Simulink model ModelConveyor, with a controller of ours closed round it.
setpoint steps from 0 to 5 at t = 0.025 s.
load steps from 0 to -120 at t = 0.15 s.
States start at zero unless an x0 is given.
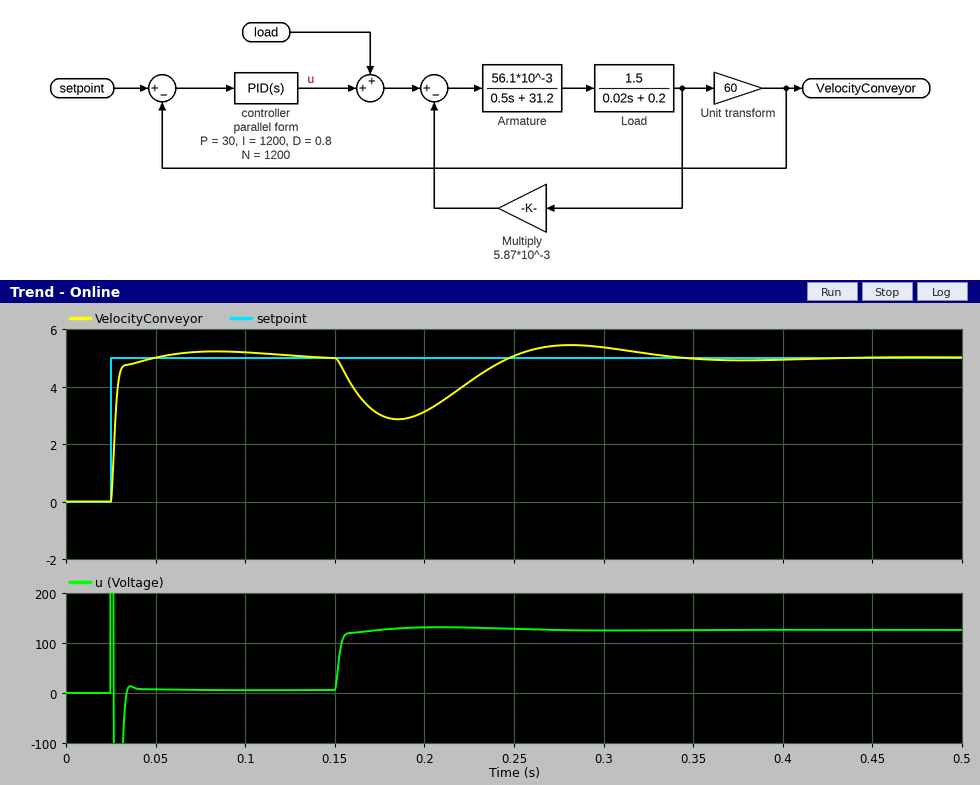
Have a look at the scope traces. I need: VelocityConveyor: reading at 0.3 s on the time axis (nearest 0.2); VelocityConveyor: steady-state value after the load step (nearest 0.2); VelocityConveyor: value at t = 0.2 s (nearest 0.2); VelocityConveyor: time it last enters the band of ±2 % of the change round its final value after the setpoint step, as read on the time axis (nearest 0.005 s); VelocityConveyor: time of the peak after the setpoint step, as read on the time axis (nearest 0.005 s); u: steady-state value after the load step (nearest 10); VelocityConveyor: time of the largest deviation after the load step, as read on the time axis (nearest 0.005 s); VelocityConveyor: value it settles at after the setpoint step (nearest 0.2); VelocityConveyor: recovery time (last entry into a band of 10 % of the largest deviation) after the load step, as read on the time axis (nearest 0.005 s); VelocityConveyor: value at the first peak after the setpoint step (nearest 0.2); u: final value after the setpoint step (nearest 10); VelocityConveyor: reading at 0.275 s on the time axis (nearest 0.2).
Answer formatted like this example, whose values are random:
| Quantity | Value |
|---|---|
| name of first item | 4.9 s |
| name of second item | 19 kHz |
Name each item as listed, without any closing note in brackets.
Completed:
| Quantity | Value |
|---|---|
| VelocityConveyor: reading at 0.3 s on the time axis | 5.4 |
| VelocityConveyor: steady-state value after the load step | 5.0 |
| VelocityConveyor: value at t = 0.2 s | 3.2 |
| VelocityConveyor: time it last enters the band of ±2 % of the change round its final value after the setpoint step, as read on the time axis | 0.120 s |
| VelocityConveyor: time of the peak after the setpoint step, as read on the time axis | 0.085 s |
| u: steady-state value after the load step | 130 |
| VelocityConveyor: time of the largest deviation after the load step, as read on the time axis | 0.185 s |
| VelocityConveyor: value it settles at after the setpoint step | 5.0 |
| VelocityConveyor: recovery time (last entry into a band of 10 % of the largest deviation) after the load step, as read on the time axis | 0.315 s |
| VelocityConveyor: value at the first peak after the setpoint step | 5.2 |
| u: final value after the setpoint step | 10 |
| VelocityConveyor: reading at 0.275 s on the time axis | 5.4 |
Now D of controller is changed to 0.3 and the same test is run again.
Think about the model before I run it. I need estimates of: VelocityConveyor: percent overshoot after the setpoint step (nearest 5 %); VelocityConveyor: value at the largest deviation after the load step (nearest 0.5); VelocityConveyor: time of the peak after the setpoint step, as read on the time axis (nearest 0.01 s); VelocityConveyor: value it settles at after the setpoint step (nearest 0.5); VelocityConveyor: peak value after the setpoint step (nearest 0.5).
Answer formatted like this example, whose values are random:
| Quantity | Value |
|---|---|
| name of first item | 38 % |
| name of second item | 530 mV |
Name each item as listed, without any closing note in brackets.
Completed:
| Quantity | Value |
|---|---|
| VelocityConveyor: percent overshoot after the setpoint step | 15 % |
| VelocityConveyor: value at the largest deviation after the load step | 2.0 |
| VelocityConveyor: time of the peak after the setpoint step, as read on the time axis | 0.05 s |
| VelocityConveyor: value it settles at after the setpoint step | 5.0 |
| VelocityConveyor: peak value after the setpoint step | 5.5 |
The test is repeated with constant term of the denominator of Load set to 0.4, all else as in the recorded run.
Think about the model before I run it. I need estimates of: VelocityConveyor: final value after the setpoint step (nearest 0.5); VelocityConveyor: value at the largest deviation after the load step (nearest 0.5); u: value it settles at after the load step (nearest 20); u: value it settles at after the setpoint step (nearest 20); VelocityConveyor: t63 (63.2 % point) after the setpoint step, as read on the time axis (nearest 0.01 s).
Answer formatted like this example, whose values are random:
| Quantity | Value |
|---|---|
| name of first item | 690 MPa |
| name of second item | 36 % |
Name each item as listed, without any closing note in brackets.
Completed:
| Quantity | Value |
|---|---|
| VelocityConveyor: final value after the setpoint step | 5.0 |
| VelocityConveyor: value at the largest deviation after the load step | 3.0 |
| u: value it settles at after the load step | 140 |
| u: value it settles at after the setpoint step | 20 |
| VelocityConveyor: t63 (63.2 % point) after the setpoint step, as read on the time axis | 0.03 s |
